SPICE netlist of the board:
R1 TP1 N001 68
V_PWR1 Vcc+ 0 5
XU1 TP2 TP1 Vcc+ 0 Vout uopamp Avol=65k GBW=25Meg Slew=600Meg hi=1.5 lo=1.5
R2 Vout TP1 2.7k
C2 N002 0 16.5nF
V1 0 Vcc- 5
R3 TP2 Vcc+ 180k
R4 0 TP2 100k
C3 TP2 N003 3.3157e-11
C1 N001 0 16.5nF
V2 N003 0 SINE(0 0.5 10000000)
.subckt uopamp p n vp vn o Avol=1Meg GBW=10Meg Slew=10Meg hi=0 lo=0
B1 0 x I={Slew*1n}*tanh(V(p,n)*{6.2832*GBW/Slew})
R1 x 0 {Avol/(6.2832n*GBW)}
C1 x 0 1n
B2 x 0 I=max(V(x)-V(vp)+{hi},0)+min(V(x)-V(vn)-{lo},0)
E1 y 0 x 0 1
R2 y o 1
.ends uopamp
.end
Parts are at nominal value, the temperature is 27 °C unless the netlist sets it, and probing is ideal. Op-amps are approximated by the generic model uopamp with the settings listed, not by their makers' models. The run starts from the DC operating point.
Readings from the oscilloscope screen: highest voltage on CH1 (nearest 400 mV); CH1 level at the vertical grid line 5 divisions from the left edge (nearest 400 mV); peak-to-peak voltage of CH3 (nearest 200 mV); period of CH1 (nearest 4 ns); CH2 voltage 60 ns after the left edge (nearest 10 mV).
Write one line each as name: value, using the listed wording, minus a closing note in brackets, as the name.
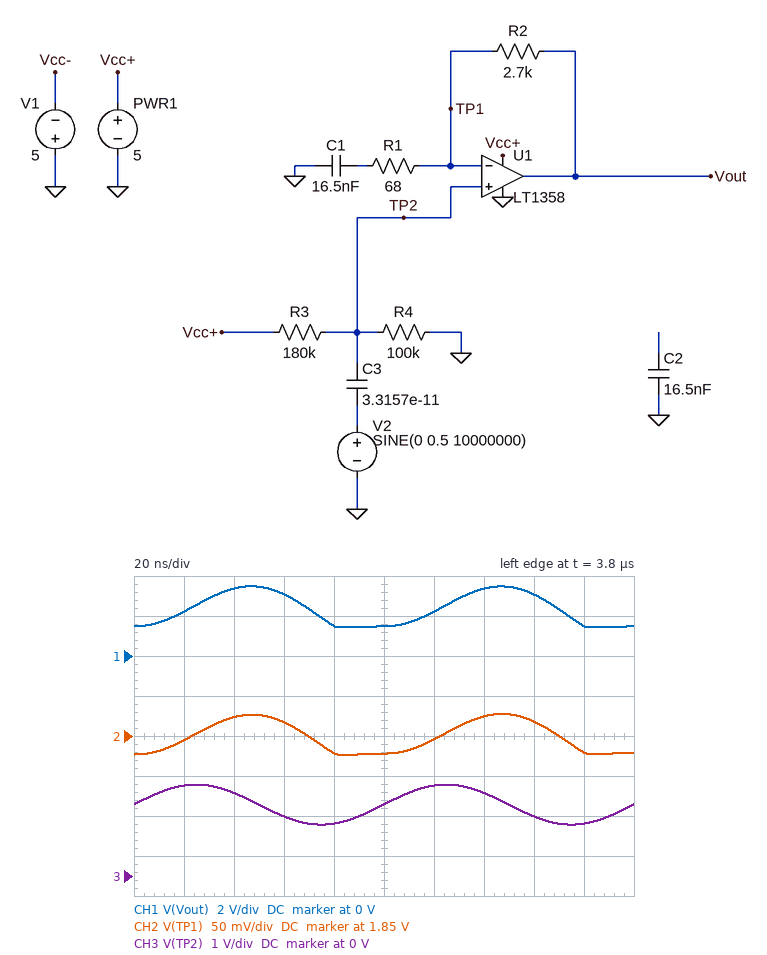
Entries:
highest voltage on CH1: 3.6 V
CH1 level at the vertical grid line 5 divisions from the left edge: 1.6 V
peak-to-peak voltage of CH3: 1.0 V
period of CH1: 100 ns
CH2 voltage 60 ns after the left edge: 1.87 V
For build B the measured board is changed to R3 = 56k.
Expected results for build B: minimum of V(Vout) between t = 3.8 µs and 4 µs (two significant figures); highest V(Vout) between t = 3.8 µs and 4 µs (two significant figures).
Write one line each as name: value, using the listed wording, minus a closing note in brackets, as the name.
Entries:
minimum of V(Vout) between t = 3.8 µs and 4 µs: 1.5 V
highest V(Vout) between t = 3.8 µs and 4 µs: 3.6 V
